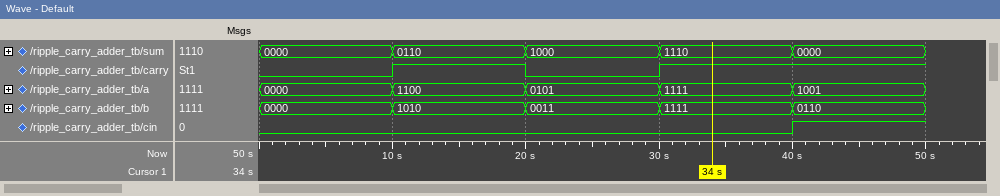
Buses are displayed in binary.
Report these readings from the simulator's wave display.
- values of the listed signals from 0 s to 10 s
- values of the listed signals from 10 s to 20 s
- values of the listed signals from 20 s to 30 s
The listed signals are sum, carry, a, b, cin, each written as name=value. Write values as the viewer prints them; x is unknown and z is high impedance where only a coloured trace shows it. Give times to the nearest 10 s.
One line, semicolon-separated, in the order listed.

sum=0000, carry=0, a=0000, b=0000, cin=0; sum=0110, carry=1, a=1100, b=1010, cin=0; sum=1000, carry=0, a=0101, b=0011, cin=0
